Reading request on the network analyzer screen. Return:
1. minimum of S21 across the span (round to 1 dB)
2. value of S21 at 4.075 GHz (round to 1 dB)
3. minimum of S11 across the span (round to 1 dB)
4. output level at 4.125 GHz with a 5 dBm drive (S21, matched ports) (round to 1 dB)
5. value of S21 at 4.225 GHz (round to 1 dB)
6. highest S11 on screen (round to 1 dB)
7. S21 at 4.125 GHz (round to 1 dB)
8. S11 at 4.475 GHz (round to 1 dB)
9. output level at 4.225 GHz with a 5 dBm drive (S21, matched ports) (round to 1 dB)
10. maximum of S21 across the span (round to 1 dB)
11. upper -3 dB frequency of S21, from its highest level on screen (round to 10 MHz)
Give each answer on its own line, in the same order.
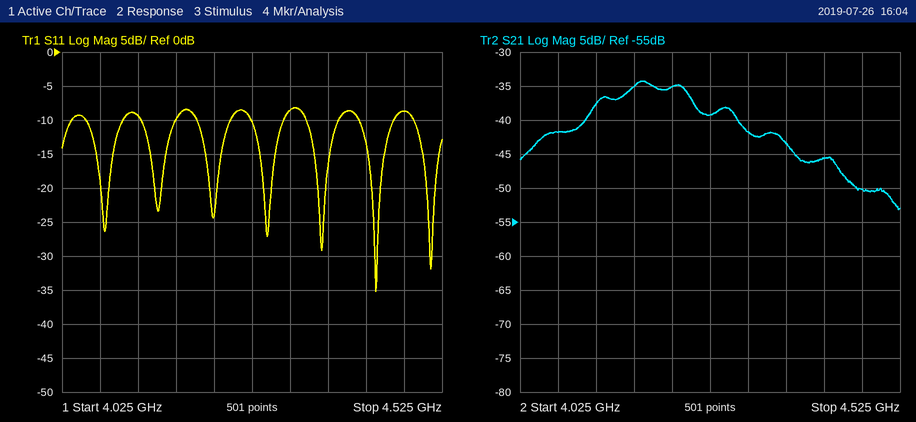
-53 dB
-42 dB
-35 dB
-33 dBm
-35 dB
-8 dB
-38 dB
-9 dB
-30 dBm
-34 dB
4.25 GHz
